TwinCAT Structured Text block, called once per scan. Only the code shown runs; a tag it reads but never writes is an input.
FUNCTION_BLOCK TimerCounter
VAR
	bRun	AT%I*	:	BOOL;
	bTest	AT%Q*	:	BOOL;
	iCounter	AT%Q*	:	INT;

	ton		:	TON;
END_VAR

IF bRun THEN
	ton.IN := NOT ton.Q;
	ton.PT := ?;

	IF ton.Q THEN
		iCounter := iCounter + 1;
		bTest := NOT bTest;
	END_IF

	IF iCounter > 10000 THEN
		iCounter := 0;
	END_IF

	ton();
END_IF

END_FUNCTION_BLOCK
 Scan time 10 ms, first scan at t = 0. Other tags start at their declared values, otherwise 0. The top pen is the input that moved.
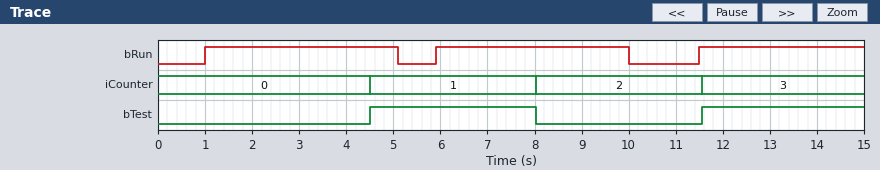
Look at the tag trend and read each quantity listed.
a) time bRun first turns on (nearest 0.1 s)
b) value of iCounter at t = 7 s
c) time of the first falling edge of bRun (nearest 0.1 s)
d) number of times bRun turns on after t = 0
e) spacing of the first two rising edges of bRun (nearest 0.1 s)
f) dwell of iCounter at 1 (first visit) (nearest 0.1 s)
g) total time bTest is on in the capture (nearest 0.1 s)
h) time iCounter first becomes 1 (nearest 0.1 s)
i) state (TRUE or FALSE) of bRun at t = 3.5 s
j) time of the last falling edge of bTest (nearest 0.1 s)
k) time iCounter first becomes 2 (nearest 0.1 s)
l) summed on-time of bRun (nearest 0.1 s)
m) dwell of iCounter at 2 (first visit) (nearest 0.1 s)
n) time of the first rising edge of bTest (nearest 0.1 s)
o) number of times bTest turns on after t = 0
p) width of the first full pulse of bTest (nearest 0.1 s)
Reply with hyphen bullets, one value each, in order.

- 1.0 s
- 1
- 5.1 s
- 3
- 4.9 s
- 3.5 s
- 7.0 s
- 4.5 s
- TRUE
- 8.0 s
- 8.0 s
- 11.7 s
- 3.5 s
- 4.5 s
- 2
- 3.5 s
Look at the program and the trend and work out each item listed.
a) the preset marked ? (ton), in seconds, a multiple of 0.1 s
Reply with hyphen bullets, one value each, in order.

- 3.5 s
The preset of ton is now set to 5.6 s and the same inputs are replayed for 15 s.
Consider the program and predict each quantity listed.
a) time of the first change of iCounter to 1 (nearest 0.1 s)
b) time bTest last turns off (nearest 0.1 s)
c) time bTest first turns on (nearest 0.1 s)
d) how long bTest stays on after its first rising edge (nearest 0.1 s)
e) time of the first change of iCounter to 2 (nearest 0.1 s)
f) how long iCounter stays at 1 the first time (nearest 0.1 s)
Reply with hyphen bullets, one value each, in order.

- 6.6 s
- 12.2 s
- 6.6 s
- 5.6 s
- 12.2 s
- 5.6 s
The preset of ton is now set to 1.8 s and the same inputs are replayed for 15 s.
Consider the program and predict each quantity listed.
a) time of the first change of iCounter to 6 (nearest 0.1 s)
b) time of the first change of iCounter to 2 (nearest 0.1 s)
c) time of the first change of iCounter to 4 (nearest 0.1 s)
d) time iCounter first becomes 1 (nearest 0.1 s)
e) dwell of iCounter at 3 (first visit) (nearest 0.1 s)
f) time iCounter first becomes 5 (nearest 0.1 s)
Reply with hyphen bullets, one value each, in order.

- 13.3 s
- 4.6 s
- 8.3 s
- 2.8 s
- 1.8 s
- 11.5 s
